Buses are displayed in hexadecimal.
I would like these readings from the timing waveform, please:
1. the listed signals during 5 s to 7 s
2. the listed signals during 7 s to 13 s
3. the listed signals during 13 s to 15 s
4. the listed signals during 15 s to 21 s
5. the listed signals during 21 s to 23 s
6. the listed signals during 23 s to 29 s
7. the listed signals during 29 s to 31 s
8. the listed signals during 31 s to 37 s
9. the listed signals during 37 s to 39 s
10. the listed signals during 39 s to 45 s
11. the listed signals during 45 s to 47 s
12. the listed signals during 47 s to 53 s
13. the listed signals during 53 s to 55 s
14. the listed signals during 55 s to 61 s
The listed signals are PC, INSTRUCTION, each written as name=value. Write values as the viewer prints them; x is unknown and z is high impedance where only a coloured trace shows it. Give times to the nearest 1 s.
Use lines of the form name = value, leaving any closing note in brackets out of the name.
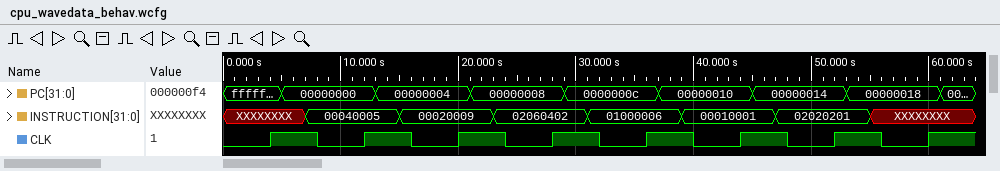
the listed signals during 5 s to 7 s = PC=00000000, INSTRUCTION=XXXXXXXX
the listed signals during 7 s to 13 s = PC=00000000, INSTRUCTION=00040005
the listed signals during 13 s to 15 s = PC=00000004, INSTRUCTION=00040005
the listed signals during 15 s to 21 s = PC=00000004, INSTRUCTION=00020009
the listed signals during 21 s to 23 s = PC=00000008, INSTRUCTION=00020009
the listed signals during 23 s to 29 s = PC=00000008, INSTRUCTION=02060402
the listed signals during 29 s to 31 s = PC=0000000c, INSTRUCTION=02060402
the listed signals during 31 s to 37 s = PC=0000000c, INSTRUCTION=01000006
the listed signals during 37 s to 39 s = PC=00000010, INSTRUCTION=01000006
the listed signals during 39 s to 45 s = PC=00000010, INSTRUCTION=00010001
the listed signals during 45 s to 47 s = PC=00000014, INSTRUCTION=00010001
the listed signals during 47 s to 53 s = PC=00000014, INSTRUCTION=02020201
the listed signals during 53 s to 55 s = PC=00000018, INSTRUCTION=02020201
the listed signals during 55 s to 61 s = PC=00000018, INSTRUCTION=XXXXXXXX
